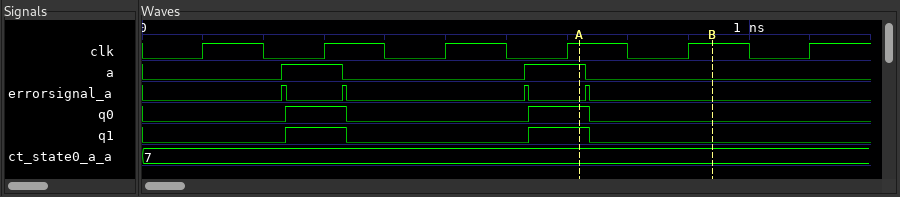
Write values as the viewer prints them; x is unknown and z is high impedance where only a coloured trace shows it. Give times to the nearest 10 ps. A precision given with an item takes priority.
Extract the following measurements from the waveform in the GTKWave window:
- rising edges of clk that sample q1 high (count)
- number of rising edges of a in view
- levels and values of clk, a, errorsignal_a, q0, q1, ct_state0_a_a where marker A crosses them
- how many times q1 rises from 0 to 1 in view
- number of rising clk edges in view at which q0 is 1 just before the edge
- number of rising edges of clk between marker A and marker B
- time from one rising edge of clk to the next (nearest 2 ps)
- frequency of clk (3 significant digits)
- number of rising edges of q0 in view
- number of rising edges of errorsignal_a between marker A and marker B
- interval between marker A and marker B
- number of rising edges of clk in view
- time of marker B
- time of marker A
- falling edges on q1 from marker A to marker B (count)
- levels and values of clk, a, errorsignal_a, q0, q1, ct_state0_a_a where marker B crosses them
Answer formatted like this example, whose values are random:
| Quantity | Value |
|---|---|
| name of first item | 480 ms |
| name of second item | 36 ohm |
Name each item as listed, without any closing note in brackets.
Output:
| Quantity | Value |
|---|---|
| rising edges of clk that sample q1 high | 2 |
| number of rising edges of a in view | 2 |
| levels and values of clk, a, errorsignal_a, q0, q1, ct_state0_a_a where marker A crosses them | clk=1, a=1, errorsignal_a=0, q0=1, q1=1, ct_state0_a_a=7 |
| how many times q1 rises from 0 to 1 in view | 2 |
| number of rising clk edges in view at which q0 is 1 just before the edge | 2 |
| number of rising edges of clk between marker A and marker B | 1 |
| time from one rising edge of clk to the next | 200 ps |
| frequency of clk | 5.00 GHz |
| number of rising edges of q0 in view | 2 |
| number of rising edges of errorsignal_a between marker A and marker B | 1 |
| interval between marker A and marker B | 220 ps |
| number of rising edges of clk in view | 6 |
| time of marker B | 940 ps |
| time of marker A | 720 ps |
| falling edges on q1 from marker A to marker B | 1 |
| levels and values of clk, a, errorsignal_a, q0, q1, ct_state0_a_a where marker B crosses them | clk=1, a=0, errorsignal_a=0, q0=0, q1=0, ct_state0_a_a=7 |
